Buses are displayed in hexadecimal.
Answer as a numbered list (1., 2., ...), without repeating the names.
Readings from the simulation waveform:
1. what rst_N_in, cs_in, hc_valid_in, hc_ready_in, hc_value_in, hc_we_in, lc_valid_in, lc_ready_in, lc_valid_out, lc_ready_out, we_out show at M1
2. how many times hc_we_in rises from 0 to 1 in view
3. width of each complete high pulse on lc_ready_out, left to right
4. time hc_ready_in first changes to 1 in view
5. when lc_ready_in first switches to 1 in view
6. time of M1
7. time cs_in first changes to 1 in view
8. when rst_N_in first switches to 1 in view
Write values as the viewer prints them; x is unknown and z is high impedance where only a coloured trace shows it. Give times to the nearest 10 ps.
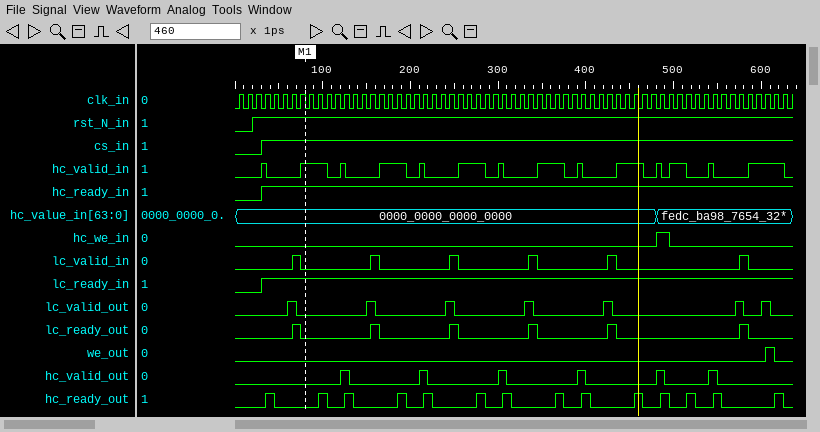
1. rst_N_in=1, cs_in=1, hc_valid_in=1, hc_ready_in=1, hc_value_in=0000_0000_0000_0000, hc_we_in=0, lc_valid_in=0, lc_ready_in=1, lc_valid_out=0, lc_ready_out=0, we_out=0
2. 1
3. 10 ps, 10 ps, 10 ps, 10 ps, 10 ps, 10 ps
4. 30 ps
5. 30 ps
6. 80 ps
7. 30 ps
8. 20 ps
